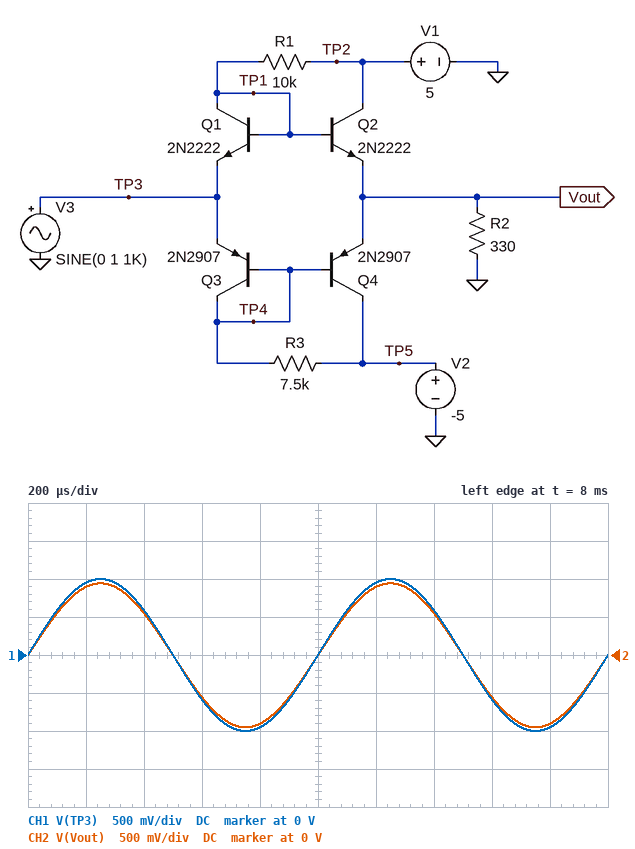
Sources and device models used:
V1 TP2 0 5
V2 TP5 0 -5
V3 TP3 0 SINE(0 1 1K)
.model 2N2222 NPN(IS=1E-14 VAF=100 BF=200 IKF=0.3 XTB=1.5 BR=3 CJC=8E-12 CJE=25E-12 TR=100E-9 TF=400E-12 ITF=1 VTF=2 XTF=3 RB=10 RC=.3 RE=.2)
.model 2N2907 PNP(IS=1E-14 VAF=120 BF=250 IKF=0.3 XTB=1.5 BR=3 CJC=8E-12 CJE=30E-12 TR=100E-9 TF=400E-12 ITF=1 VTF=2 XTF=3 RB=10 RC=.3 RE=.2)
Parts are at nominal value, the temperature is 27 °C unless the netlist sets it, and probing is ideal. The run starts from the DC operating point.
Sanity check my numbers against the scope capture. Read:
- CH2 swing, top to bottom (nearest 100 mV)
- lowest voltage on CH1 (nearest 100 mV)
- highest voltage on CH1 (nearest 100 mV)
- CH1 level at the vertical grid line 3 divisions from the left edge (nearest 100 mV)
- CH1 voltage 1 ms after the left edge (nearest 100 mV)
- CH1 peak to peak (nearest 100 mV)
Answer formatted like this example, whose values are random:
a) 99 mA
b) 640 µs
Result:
a) 1.9 V
b) -1.0 V
c) 1.0 V
d) -600 mV
e) 0 V
f) 2.0 V
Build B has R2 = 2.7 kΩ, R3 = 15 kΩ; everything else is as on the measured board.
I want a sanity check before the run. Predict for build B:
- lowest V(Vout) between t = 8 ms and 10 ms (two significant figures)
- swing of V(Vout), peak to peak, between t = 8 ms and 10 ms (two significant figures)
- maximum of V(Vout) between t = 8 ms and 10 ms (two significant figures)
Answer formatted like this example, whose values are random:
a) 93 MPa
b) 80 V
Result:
a) -980 mV
b) 2.0 V
c) 990 mV
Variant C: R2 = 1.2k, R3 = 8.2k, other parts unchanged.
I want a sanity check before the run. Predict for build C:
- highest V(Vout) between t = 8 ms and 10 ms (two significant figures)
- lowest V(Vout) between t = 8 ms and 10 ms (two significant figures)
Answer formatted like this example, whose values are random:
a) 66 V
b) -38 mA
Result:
a) 970 mV
b) -980 mV
